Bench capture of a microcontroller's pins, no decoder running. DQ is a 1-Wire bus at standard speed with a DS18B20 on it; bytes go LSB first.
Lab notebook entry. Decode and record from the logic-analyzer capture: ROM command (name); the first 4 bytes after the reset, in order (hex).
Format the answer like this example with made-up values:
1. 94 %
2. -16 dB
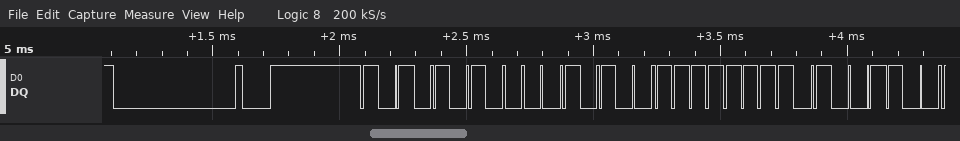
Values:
1. Match ROM
2. 55 28 FF 32
